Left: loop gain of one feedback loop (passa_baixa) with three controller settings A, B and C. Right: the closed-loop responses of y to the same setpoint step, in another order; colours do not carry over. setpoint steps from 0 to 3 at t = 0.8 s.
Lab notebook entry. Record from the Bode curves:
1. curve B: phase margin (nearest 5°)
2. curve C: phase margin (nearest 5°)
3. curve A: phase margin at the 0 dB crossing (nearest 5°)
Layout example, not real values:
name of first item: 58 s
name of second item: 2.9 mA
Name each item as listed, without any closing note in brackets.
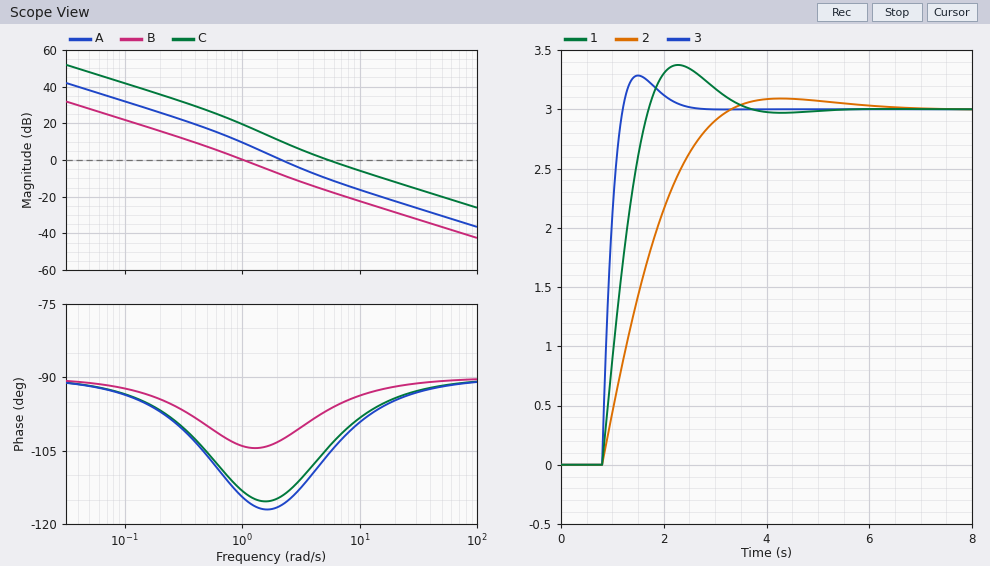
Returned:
curve B: phase margin: 75°
curve C: phase margin: 75°
curve A: phase margin at the 0 dB crossing: 65°
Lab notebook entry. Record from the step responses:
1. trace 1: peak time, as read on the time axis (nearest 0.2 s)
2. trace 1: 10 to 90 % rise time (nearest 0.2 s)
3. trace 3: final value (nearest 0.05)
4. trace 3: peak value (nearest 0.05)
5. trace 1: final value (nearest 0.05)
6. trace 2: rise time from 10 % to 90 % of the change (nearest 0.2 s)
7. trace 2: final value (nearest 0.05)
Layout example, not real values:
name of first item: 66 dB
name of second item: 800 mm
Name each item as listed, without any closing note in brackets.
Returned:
trace 1: peak time, as read on the time axis: 2.2 s
trace 1: 10 to 90 % rise time: 0.6 s
trace 3: final value: 3.00
trace 3: peak value: 3.30
trace 1: final value: 3.00
trace 2: rise time from 10 % to 90 % of the change: 1.6 s
trace 2: final value: 3.00
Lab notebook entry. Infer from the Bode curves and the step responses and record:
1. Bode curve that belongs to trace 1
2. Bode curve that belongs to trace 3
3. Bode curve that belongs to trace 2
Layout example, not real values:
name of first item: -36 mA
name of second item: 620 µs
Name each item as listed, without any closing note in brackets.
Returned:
Bode curve that belongs to trace 1: A
Bode curve that belongs to trace 3: C
Bode curve that belongs to trace 2: B
